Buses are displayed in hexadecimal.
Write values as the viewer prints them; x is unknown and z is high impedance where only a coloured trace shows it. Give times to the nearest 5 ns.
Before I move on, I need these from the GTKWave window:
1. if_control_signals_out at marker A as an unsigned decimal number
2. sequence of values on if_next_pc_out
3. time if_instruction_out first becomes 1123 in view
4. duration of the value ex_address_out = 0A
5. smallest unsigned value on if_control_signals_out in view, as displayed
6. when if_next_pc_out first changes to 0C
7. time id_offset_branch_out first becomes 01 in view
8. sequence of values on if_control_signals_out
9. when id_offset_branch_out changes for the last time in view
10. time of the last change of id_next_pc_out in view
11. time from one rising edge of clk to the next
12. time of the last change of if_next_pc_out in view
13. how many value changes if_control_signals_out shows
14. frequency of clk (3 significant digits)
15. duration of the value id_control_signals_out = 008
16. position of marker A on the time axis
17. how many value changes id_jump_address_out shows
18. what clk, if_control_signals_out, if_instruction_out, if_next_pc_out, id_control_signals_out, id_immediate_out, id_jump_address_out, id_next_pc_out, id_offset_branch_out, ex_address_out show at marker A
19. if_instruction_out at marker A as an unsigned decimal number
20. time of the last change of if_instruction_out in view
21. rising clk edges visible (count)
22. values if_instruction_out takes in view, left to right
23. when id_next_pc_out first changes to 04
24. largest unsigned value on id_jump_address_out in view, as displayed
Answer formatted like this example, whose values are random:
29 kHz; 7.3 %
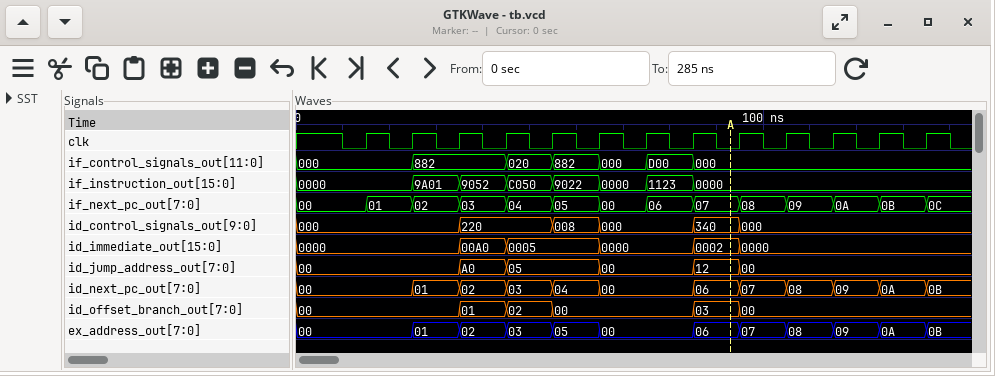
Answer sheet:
0; 00, 01, 02, 03, 04, 05, 00, 06, 07, 08, 09, 0A, 0B, 0C; 75 ns; 10 ns; 000; 135 ns; 35 ns; 000, 882, 020, 882, 000, D00, 000; 95 ns; 135 ns; 10 ns; 135 ns; 6; 100 MHz; 10 ns; 95 ns; 5; clk=0, if_control_signals_out=000, if_instruction_out=0000, if_next_pc_out=07, id_control_signals_out=340, id_immediate_out=0002, id_jump_address_out=12, id_next_pc_out=06, id_offset_branch_out=03, ex_address_out=06; 0; 85 ns; 13; 0000, 9A01, 9052, C050, 9022, 0000, 1123, 0000; 55 ns; A0
